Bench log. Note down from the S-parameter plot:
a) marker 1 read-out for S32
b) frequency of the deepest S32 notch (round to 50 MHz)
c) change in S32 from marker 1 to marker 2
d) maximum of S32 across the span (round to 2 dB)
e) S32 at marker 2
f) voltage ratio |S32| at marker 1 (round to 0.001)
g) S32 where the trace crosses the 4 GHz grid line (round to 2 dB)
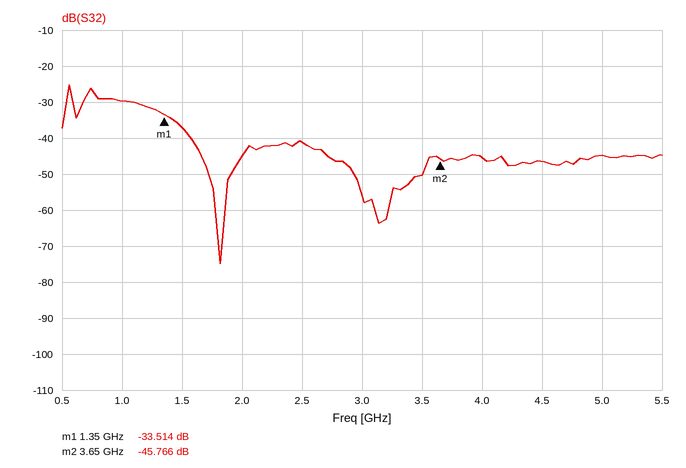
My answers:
-33.514 dB
1.80 GHz
-12.252 dB
-26 dB
-45.766 dB
0.021
-46 dB
